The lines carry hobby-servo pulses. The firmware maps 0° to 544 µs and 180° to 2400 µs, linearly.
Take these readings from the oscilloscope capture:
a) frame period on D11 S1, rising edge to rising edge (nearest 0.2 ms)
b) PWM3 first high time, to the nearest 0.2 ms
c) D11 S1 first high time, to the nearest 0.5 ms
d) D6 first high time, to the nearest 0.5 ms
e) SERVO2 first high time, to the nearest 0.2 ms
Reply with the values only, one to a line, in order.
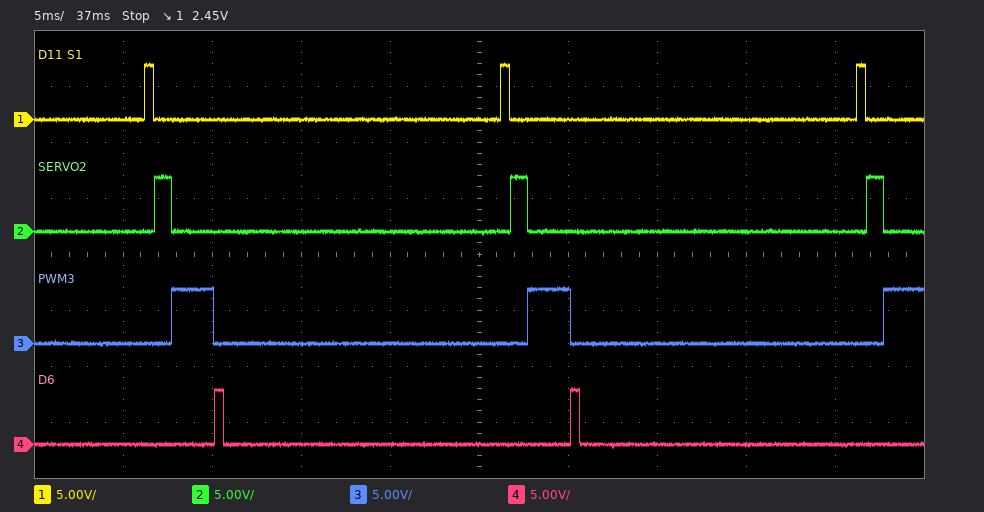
20.0 ms
2.4 ms
0.5 ms
0.5 ms
1.0 ms
